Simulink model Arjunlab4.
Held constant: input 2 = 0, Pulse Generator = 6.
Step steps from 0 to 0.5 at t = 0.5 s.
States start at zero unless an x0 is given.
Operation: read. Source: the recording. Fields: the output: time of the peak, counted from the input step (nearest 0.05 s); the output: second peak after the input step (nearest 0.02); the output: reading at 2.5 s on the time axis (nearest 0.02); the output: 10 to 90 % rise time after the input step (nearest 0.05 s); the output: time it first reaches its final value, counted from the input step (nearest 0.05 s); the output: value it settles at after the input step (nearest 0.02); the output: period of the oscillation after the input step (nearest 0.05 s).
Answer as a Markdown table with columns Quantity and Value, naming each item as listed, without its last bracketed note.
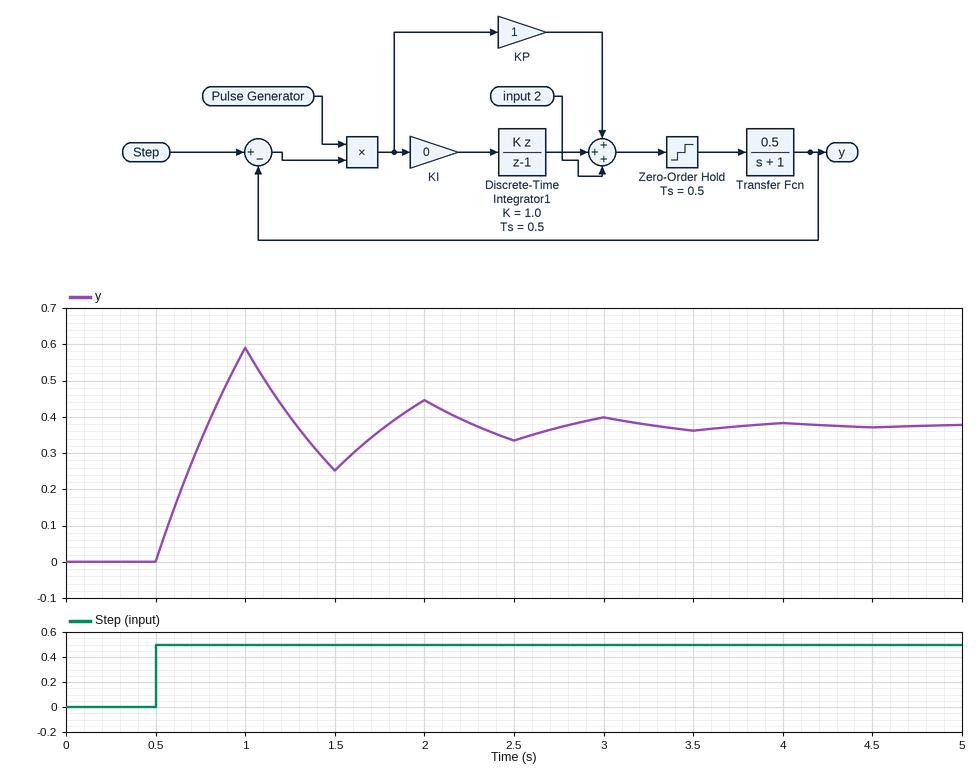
| Quantity | Value |
|---|---|
| the output: time of the peak, counted from the input step | 0.50 s |
| the output: second peak after the input step | 0.44 |
| the output: reading at 2.5 s on the time axis | 0.34 |
| the output: 10 to 90 % rise time after the input step | 0.25 s |
| the output: time it first reaches its final value, counted from the input step | 0.30 s |
| the output: value it settles at after the input step | 0.38 |
| the output: period of the oscillation after the input step | 1.00 s |
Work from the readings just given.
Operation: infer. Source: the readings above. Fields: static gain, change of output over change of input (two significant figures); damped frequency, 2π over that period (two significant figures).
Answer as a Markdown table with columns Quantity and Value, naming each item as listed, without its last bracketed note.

| Quantity | Value |
|---|---|
| static gain, change of output over change of input | 0.76 |
| damped frequency, 2π over that period | 6.3 rad/s |
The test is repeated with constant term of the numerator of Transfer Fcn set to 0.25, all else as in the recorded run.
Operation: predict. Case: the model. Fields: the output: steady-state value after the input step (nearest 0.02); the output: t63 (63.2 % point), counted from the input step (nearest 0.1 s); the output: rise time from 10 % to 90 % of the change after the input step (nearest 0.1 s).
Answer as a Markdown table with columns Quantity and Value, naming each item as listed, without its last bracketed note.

| Quantity | Value |
|---|---|
| the output: steady-state value after the input step | 0.30 |
| the output: t63 (63.2 % point), counted from the input step | 0.3 s |
| the output: rise time from 10 % to 90 % of the change after the input step | 0.4 s |
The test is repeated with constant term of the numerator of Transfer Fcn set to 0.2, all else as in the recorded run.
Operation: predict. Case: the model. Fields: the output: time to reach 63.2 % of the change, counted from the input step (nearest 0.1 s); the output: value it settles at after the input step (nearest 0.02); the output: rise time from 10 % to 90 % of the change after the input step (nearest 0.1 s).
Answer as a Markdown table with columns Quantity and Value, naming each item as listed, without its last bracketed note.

| Quantity | Value |
|---|---|
| the output: time to reach 63.2 % of the change, counted from the input step | 0.3 s |
| the output: value it settles at after the input step | 0.28 |
| the output: rise time from 10 % to 90 % of the change after the input step | 0.6 s |
